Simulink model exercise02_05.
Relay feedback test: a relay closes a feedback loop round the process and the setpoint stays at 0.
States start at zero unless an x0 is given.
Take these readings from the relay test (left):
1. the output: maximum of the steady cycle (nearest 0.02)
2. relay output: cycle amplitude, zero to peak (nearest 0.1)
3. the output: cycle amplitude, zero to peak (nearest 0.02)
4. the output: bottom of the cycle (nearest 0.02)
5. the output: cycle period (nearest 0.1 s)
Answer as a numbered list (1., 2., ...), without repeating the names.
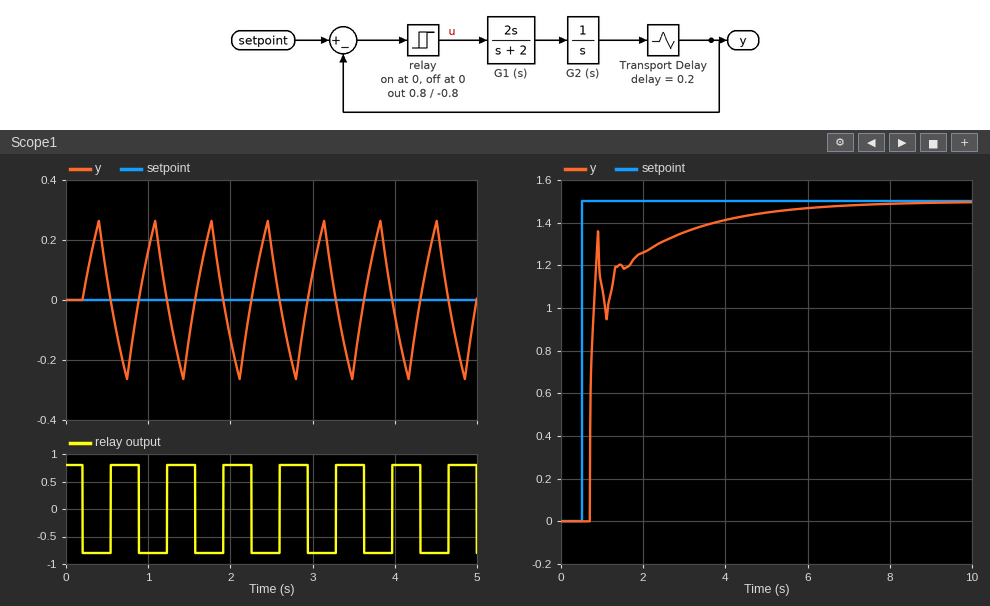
1. 0.26
2. 0.8
3. 0.26
4. -0.26
5. 0.7 s
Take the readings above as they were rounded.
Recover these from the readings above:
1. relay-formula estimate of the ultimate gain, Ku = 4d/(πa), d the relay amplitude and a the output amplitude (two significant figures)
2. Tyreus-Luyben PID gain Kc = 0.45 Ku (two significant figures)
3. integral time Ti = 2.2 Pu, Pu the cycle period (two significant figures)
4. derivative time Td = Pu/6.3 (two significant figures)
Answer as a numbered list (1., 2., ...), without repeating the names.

1. 3.9
2. 1.8
3. 1.5 s
4. 0.11 s
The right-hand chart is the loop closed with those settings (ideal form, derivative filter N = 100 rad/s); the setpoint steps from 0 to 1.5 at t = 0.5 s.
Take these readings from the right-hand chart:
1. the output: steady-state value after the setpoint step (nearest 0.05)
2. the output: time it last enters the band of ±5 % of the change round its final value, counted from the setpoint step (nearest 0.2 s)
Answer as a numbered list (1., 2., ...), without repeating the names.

1. 1.50
2. 3.8 s
